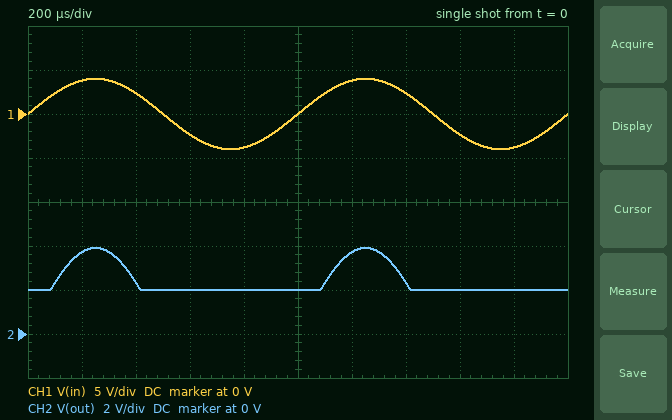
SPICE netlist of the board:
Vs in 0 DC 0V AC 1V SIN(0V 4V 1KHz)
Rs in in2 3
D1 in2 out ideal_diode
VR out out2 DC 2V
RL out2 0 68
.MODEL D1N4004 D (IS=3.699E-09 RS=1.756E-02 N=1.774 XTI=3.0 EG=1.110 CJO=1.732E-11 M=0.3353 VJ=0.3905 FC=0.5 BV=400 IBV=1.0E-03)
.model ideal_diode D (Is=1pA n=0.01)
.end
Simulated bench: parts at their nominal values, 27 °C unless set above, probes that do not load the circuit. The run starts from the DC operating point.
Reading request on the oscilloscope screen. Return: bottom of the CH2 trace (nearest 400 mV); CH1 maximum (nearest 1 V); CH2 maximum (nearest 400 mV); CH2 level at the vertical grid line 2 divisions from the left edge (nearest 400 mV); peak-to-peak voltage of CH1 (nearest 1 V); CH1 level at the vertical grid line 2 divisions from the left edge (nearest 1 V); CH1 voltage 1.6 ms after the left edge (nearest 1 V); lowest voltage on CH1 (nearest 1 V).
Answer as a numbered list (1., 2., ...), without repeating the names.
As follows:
1. 2.0 V
2. 4 V
3. 4.0 V
4. 2.4 V
5. 8 V
6. 2 V
7. -2 V
8. -4 V
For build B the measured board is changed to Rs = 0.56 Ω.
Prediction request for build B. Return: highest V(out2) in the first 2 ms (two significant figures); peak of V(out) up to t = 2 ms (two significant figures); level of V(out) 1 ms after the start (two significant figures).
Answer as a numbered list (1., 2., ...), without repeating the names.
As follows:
1. 2.0 V
2. 4.0 V
3. 2.0 V
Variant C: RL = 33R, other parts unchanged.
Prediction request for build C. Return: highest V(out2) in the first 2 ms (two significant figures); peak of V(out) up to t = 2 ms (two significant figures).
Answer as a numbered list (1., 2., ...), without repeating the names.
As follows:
1. 1.8 V
2. 3.8 V
